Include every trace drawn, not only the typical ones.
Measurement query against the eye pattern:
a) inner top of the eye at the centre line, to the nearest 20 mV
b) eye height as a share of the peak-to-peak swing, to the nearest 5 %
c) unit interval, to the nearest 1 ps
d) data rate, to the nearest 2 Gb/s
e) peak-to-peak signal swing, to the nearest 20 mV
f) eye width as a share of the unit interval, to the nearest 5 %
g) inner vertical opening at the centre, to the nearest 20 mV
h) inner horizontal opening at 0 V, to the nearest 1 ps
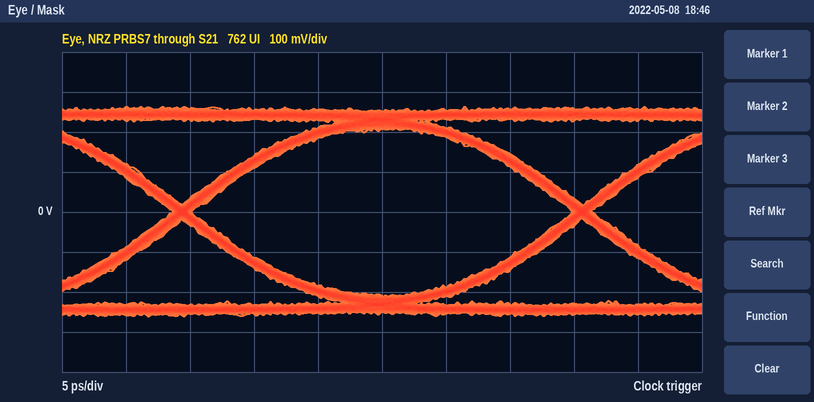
200 mV
80 %
31 ps
32 Gb/s
520 mV
95 %
420 mV
30 ps
